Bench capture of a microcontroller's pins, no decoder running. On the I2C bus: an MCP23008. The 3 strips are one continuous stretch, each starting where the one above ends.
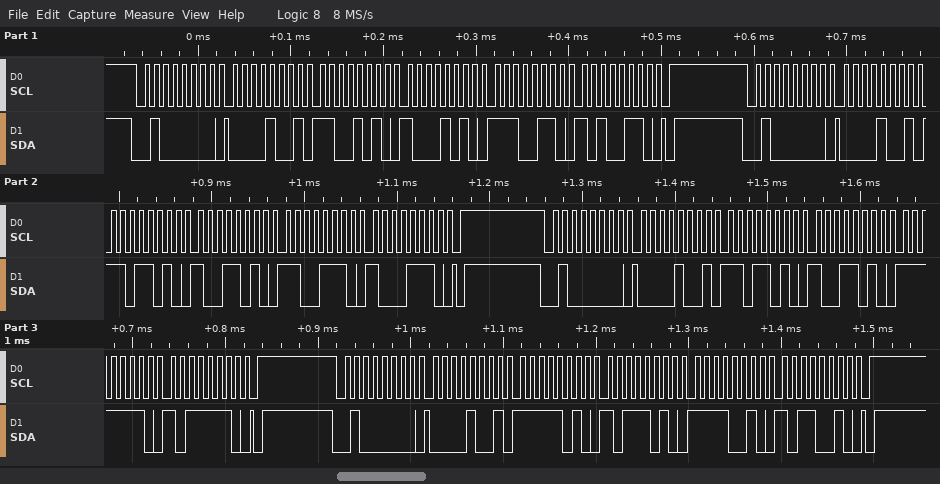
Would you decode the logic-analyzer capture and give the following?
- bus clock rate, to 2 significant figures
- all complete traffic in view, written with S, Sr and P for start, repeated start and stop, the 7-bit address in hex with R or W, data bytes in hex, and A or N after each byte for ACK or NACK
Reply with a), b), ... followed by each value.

a) 100 kHz
b) S 20W A 09 A CA A 8A A E6 A A6 A P S 20W A 09 A DA A 9A A CE A 8E A P S 20W A 09 A DA A 9A A FE A BE A P S 20W A 09 A FA A BA A F2 A B2 A P
